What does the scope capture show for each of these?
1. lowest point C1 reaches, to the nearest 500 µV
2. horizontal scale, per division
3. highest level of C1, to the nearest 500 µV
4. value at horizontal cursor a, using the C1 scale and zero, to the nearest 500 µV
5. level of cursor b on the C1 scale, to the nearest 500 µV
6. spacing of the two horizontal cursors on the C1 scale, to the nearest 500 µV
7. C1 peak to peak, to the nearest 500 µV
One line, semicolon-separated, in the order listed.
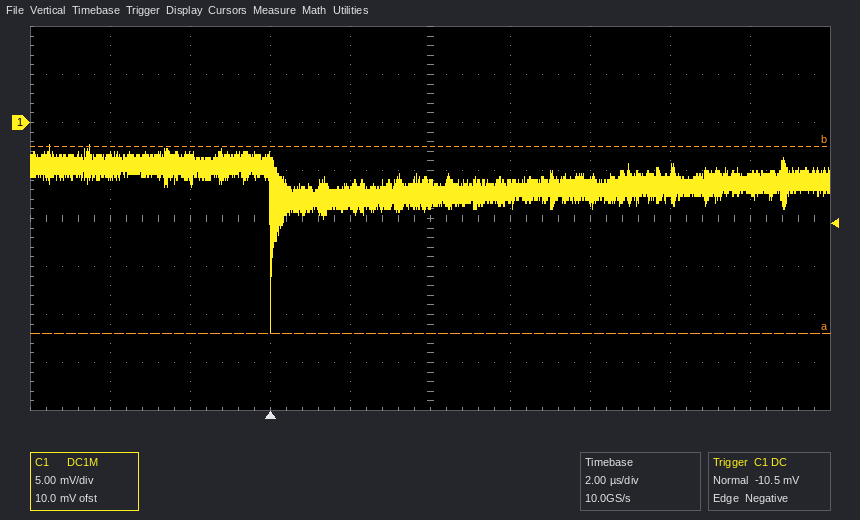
-22.0 mV; 2 µs; -2.5 mV; -22.0 mV; -2.5 mV; 19.5 mV; 19.5 mV
